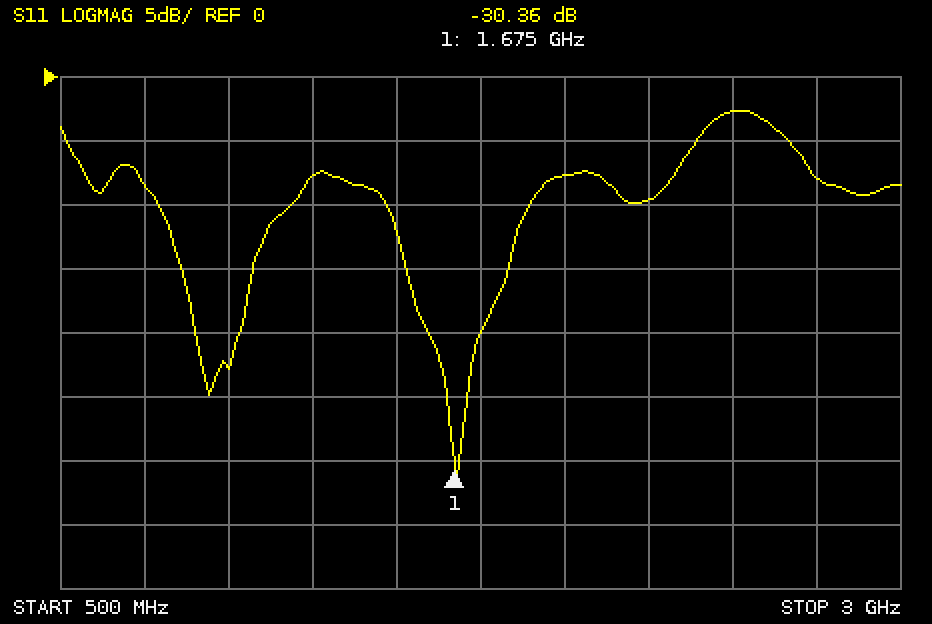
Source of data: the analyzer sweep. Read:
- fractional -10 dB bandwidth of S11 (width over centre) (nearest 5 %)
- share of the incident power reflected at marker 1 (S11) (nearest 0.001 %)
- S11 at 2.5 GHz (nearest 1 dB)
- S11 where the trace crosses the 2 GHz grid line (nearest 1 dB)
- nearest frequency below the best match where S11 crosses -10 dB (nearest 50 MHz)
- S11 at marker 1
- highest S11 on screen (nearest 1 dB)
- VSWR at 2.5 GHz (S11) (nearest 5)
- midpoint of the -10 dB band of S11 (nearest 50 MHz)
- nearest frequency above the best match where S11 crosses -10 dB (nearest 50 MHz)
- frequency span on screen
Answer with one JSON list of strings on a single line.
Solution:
["25 %", "0.092 %", "-3 dB", "-8 dB", "1.45 GHz", "-30.36 dB", "-3 dB", "5", "1.70 GHz", "1.90 GHz", "2.5 GHz"]
